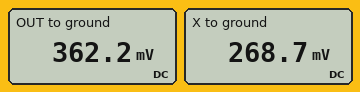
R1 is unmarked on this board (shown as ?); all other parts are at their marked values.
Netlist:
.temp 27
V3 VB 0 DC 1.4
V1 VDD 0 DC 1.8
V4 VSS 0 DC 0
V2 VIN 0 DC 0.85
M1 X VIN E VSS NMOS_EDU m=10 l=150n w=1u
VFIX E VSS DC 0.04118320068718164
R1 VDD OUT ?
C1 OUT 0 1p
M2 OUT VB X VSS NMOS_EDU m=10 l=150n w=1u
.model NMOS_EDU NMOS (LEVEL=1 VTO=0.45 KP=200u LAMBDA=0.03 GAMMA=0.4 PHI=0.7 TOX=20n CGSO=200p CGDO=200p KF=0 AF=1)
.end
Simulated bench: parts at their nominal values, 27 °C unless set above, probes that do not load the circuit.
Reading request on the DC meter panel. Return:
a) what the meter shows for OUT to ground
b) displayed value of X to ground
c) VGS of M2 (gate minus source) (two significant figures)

362.2 mV
268.7 mV
1.1 V
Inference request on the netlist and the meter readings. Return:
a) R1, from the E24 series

2 kΩ
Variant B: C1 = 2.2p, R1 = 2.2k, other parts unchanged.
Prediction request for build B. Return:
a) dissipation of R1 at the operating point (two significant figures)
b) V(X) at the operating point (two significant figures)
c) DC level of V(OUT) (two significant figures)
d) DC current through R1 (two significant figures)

990 µW
240 mV
320 mV
670 µA
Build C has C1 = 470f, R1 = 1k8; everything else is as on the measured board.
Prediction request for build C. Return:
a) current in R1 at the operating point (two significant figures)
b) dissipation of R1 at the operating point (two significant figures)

770 µA
1.1 mW
